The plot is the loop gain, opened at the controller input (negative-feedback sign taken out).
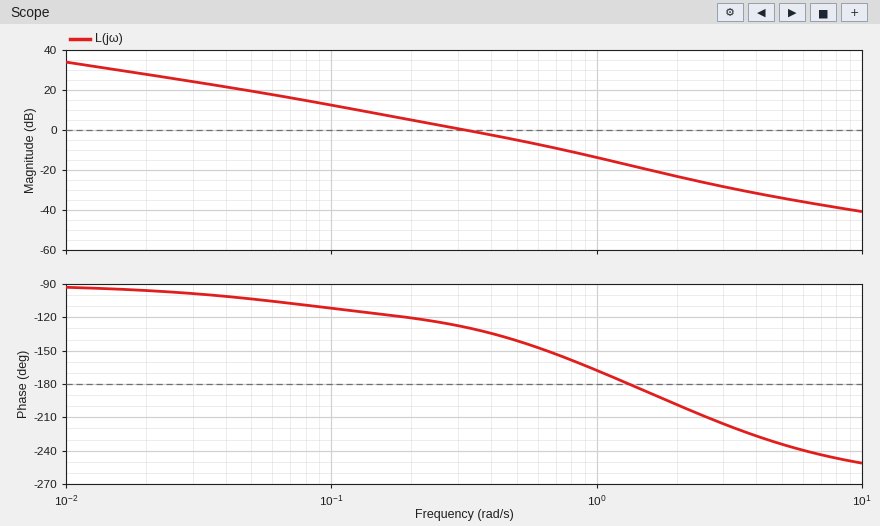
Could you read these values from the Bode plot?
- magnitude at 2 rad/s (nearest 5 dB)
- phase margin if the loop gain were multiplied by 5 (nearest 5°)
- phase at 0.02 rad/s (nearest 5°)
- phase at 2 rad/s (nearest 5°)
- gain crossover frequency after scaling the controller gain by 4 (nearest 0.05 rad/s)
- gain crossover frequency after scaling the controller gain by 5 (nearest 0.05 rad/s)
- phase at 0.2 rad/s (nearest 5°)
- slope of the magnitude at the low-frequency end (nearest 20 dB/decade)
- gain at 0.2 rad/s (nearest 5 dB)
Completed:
-25 dB
10°
-95°
-200°
0.90 rad/s
1.00 rad/s
-120°
-20 dB/decade
5 dB
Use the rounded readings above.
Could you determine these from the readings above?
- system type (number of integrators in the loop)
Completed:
1
